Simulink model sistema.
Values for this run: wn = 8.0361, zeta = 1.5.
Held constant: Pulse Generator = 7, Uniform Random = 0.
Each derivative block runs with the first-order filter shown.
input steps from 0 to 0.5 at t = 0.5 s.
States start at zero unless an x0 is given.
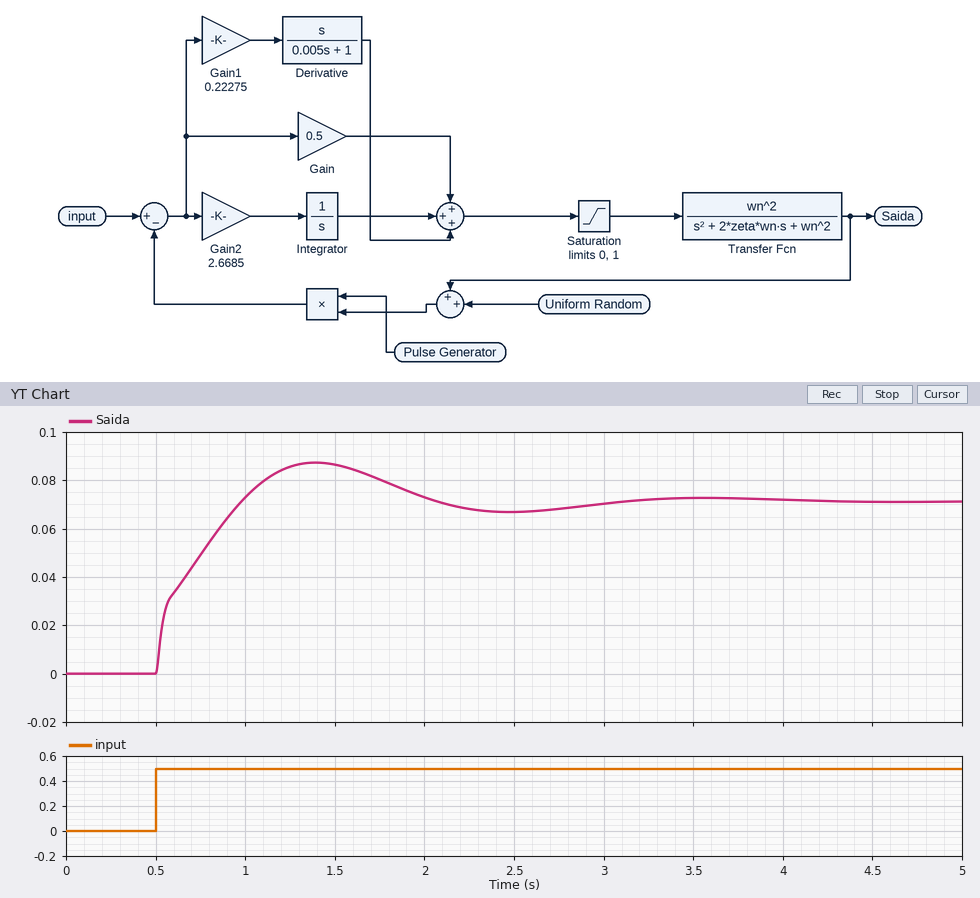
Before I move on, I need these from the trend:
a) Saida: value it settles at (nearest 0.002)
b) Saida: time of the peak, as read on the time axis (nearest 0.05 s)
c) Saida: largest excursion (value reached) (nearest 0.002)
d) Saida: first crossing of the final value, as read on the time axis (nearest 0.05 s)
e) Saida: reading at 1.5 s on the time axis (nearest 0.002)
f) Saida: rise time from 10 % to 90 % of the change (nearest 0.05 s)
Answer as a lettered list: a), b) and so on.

a) 0.072
b) 1.40 s
c) 0.088
d) 1.00 s
e) 0.086
f) 0.40 s
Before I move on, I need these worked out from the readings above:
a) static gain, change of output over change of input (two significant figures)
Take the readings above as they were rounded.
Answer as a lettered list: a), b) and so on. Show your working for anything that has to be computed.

a) (0.072 - 0) / (0.5 - 0) = 0.14
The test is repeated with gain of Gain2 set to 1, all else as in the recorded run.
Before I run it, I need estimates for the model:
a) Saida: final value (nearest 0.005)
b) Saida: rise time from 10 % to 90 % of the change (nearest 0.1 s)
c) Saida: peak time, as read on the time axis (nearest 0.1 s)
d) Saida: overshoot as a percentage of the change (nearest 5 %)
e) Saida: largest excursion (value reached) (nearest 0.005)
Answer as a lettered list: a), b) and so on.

a) 0.070
b) 0.6 s
c) 2.0 s
d) 10 %
e) 0.080
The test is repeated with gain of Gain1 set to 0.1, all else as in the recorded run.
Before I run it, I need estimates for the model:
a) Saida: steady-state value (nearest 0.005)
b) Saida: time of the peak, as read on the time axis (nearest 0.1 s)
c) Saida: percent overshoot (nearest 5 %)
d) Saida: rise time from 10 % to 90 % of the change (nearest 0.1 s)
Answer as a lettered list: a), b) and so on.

a) 0.070
b) 1.1 s
c) 20 %
d) 0.3 s
